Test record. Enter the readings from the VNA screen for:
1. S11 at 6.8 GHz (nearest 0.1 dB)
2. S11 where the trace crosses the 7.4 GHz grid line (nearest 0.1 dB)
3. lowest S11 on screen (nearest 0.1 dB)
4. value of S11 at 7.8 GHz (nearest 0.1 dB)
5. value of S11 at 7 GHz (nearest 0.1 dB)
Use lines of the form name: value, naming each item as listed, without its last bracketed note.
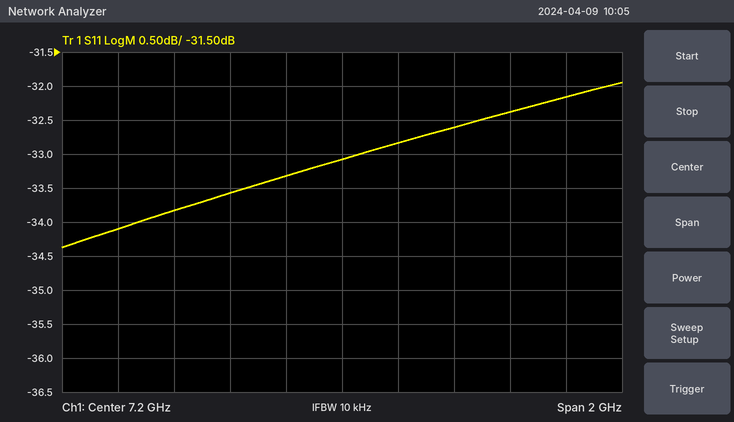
S11 at 6.8 GHz: -33.6 dB
S11 where the trace crosses the 7.4 GHz grid line: -32.8 dB
lowest S11 on screen: -34.4 dB
value of S11 at 7.8 GHz: -32.4 dB
value of S11 at 7 GHz: -33.3 dB
